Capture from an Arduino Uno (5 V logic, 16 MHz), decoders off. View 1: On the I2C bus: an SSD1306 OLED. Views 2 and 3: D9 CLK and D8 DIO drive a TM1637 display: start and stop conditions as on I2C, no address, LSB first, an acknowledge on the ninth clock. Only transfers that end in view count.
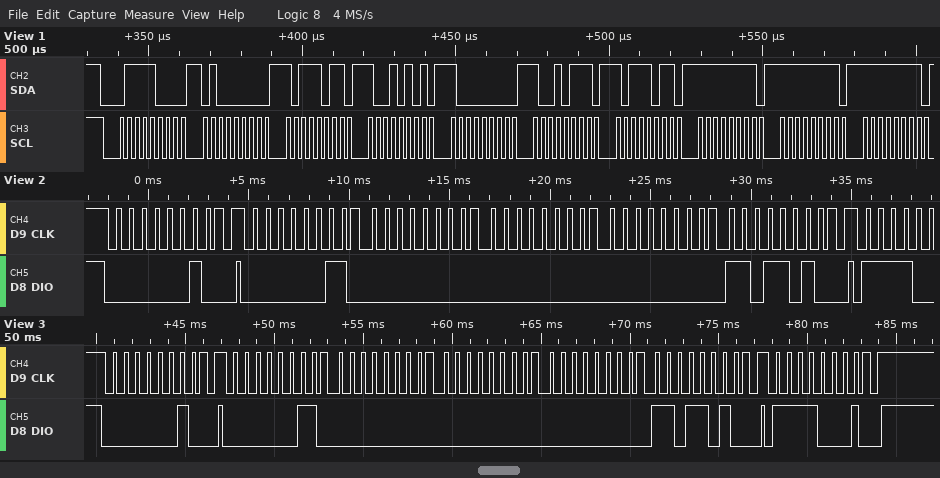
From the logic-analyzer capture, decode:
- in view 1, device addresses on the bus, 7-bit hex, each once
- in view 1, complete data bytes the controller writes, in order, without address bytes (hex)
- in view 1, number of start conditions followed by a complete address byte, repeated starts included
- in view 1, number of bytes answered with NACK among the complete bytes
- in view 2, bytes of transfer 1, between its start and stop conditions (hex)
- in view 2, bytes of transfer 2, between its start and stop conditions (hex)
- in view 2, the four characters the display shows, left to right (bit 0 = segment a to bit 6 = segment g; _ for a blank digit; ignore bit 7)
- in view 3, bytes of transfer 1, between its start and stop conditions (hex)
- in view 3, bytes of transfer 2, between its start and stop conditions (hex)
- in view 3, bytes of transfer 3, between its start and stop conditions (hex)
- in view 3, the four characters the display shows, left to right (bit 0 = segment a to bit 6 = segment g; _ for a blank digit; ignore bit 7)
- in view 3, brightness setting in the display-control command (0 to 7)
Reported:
0x3C
40 BB 95 80 97 BB FF FF FF
1
0
40
C0 00 00 00 5B
___2
40
C0 00 00 00 5B
8F
___2
7
